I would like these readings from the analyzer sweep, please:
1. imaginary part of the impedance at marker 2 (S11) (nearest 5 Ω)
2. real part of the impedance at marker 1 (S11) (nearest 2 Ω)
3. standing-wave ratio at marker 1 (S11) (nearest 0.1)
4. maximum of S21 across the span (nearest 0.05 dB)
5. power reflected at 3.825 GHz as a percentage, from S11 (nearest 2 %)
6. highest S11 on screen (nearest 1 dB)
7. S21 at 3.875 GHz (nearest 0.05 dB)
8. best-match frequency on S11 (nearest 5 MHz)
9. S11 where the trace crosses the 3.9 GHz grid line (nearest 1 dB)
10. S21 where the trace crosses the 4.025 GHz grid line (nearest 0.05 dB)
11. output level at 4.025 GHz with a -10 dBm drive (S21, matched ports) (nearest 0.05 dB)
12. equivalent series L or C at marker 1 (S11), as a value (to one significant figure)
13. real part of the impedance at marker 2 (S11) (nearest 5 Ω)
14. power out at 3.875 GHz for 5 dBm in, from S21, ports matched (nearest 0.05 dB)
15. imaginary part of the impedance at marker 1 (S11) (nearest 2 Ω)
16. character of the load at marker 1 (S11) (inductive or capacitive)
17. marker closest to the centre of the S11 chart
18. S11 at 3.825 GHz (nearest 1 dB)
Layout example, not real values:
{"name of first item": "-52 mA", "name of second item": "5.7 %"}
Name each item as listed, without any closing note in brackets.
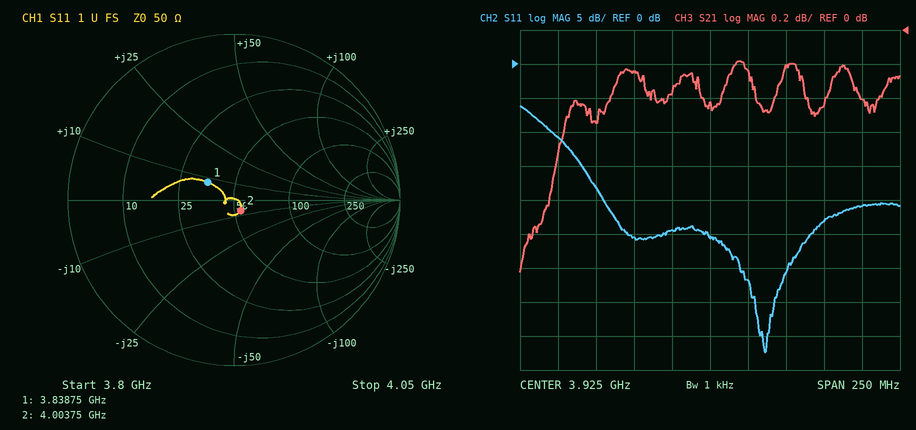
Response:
{"imaginary part of the impedance at marker 2 (S11)": "-5 Ω", "real part of the impedance at marker 1 (S11)": "36 Ω", "standing-wave ratio at marker 1 (S11)": "1.5", "maximum of S21 across the span": "-0.20 dB", "power reflected at 3.825 GHz as a percentage, from S11": "8 %", "highest S11 on screen": "-6 dB", "S21 at 3.875 GHz": "-0.25 dB", "best-match frequency on S11": "3.960 GHz", "S11 where the trace crosses the 3.9 GHz grid line": "-24 dB", "S21 where the trace crosses the 4.025 GHz grid line": "-0.40 dB", "output level at 4.025 GHz with a -10 dBm drive (S21, matched ports)": "-10.40 dBm", "equivalent series L or C at marker 1 (S11), as a value": "300 pH", "real part of the impedance at marker 2 (S11)": "55 Ω", "power out at 3.875 GHz for 5 dBm in, from S21, ports matched": "4.75 dBm", "imaginary part of the impedance at marker 1 (S11)": "+8 Ω", "character of the load at marker 1 (S11)": "inductive", "marker closest to the centre of the S11 chart": "marker 2", "S11 at 3.825 GHz": "-11 dB"}
